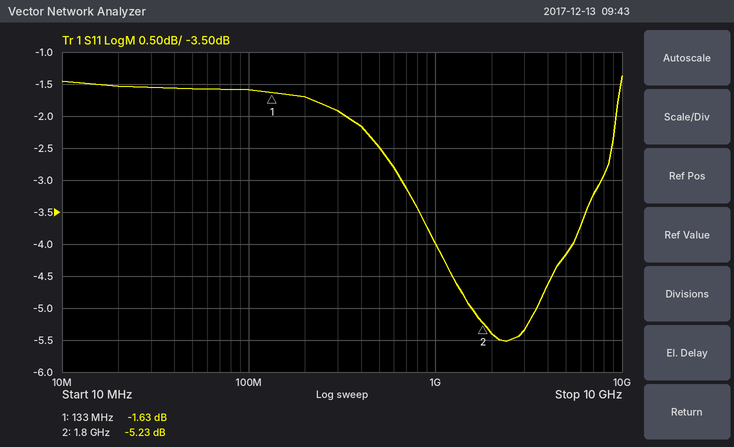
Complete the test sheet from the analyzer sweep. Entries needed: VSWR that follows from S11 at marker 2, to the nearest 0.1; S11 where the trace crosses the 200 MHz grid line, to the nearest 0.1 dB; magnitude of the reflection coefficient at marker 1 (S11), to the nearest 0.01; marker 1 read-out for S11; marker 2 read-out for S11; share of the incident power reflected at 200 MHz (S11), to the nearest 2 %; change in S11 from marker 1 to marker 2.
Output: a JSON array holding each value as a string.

["3.4", "-1.7 dB", "0.83", "-1.63 dB", "-5.23 dB", "68 %", "-3.60 dB"]
